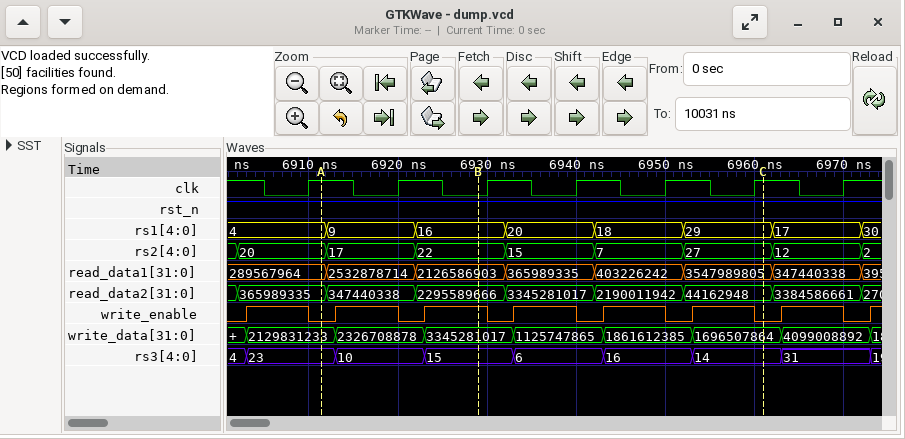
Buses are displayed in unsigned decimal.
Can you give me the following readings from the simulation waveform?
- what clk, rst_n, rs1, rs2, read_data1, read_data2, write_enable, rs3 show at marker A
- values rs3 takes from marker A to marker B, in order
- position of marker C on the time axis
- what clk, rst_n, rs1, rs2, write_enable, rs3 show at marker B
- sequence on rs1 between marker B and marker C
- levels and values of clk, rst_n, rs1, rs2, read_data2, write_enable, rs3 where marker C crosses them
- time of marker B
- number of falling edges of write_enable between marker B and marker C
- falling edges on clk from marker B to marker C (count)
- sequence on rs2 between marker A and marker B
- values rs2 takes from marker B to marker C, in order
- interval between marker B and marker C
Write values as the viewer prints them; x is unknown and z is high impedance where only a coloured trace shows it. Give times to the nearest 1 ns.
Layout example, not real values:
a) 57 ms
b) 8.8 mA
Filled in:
a) clk=1, rst_n=1, rs1=4, rs2=20, read_data1=289567964, read_data2=365989335, write_enable=0, rs3=23
b) 23, 10, 15
c) 6961 ns
d) clk=0, rst_n=1, rs1=16, rs2=22, write_enable=1, rs3=15
e) 16, 20, 18, 29
f) clk=1, rst_n=1, rs1=29, rs2=27, read_data2=44162948, write_enable=0, rs3=14
g) 6929 ns
h) 4
i) 3
j) 20, 17, 22
k) 22, 15, 7, 27
l) 32 ns
